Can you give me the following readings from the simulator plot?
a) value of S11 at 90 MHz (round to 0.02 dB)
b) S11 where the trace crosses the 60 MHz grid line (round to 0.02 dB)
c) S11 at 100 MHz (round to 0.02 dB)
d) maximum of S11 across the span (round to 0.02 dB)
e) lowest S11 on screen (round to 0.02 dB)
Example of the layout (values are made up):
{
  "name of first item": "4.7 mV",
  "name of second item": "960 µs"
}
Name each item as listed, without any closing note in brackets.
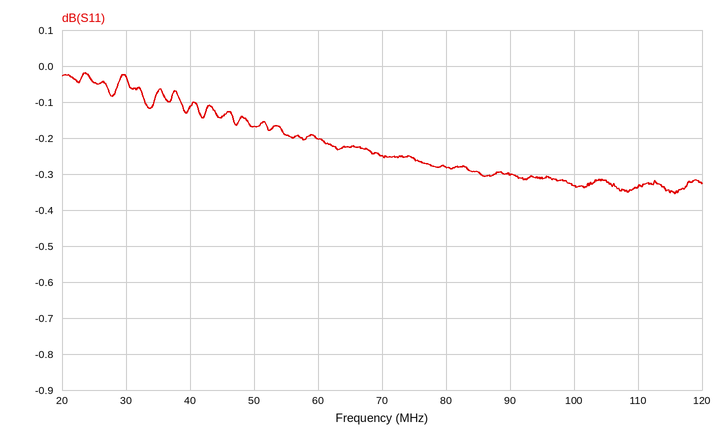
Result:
{
  "value of S11 at 90 MHz": "-0.30 dB",
  "S11 where the trace crosses the 60 MHz grid line": "-0.20 dB",
  "S11 at 100 MHz": "-0.34 dB",
  "maximum of S11 across the span": "-0.02 dB",
  "lowest S11 on screen": "-0.36 dB"
}
